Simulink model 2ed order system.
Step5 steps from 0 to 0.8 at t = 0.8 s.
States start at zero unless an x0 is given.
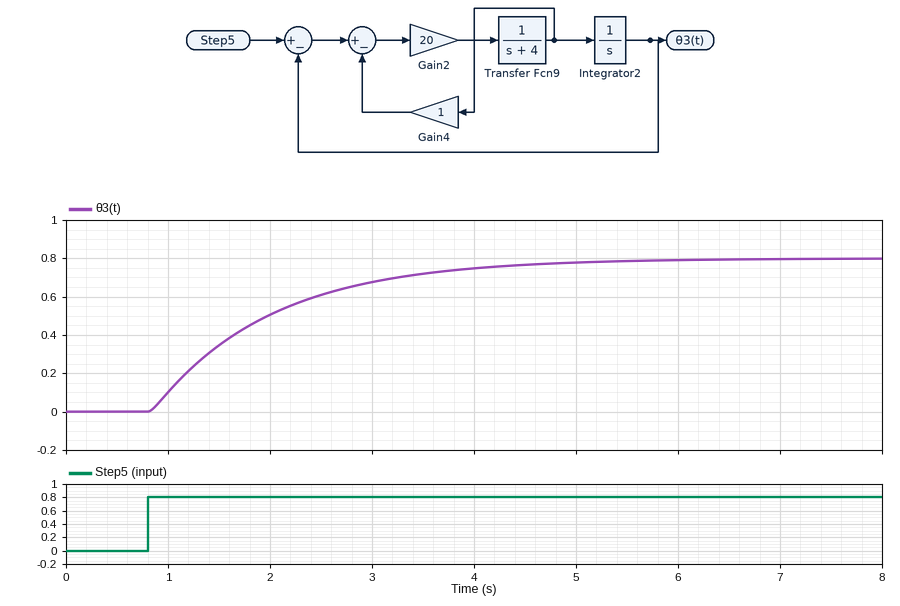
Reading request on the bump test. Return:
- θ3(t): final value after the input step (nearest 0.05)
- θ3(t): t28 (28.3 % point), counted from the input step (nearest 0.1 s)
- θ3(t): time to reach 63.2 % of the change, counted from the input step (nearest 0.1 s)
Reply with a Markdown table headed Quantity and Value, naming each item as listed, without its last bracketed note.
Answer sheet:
| Quantity | Value |
|---|---|
| θ3(t): final value after the input step | 0.80 |
| θ3(t): t28 (28.3 % point), counted from the input step | 0.4 s |
| θ3(t): time to reach 63.2 % of the change, counted from the input step | 1.2 s |
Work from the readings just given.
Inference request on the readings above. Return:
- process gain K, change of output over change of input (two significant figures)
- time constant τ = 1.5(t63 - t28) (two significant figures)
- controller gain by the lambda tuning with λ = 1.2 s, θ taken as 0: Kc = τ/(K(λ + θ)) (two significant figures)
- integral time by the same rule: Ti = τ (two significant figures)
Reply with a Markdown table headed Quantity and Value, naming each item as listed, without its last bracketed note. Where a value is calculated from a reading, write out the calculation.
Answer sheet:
| Quantity | Value |
|---|---|
| process gain K, change of output over change of input | (0.8 - 0) / 0.8 = 1.0 |
| time constant τ = 1.5(t63 - t28) | 1.5 × (1.2 - 0.4) = 1.2 s |
| controller gain by the lambda tuning with λ = 1.2 s, θ taken as 0: Kc = τ/(K(λ + θ)) | 1.2 / (1 × (1.2 + 0)) = 1.0 |
| integral time by the same rule: Ti = τ | 1.2 s |
